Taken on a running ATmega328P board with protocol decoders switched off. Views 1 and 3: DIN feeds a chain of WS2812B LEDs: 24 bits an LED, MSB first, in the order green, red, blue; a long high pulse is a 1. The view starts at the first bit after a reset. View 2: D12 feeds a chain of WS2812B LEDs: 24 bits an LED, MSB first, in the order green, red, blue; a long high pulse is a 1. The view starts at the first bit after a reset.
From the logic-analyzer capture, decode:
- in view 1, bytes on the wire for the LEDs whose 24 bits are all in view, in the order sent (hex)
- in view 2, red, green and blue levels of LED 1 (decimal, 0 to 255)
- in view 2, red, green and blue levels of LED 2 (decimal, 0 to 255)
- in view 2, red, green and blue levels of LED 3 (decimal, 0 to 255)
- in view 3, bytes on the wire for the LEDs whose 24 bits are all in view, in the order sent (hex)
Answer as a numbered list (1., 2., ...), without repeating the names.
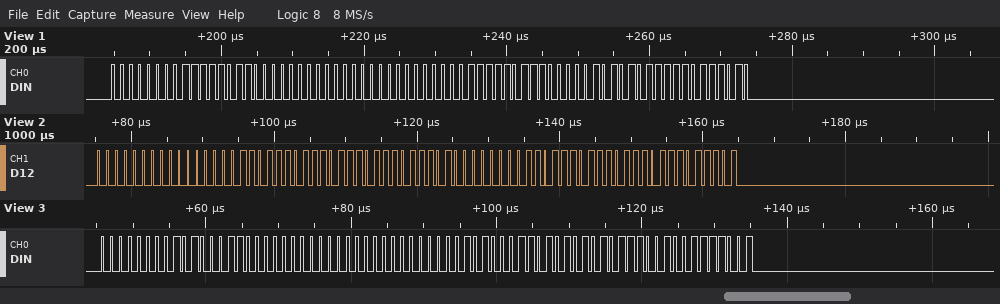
1. 00 FB 00 00 00 FB 82 AF BA
2. 0, 0, 221
3. 221, 221, 0
4. 221, 221, 221
5. 00 A3 00 00 00 A3 55 72 79
